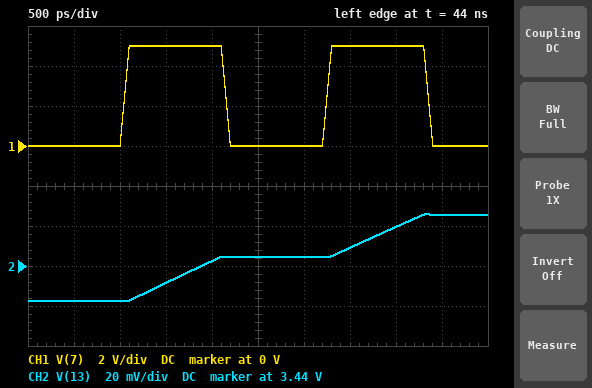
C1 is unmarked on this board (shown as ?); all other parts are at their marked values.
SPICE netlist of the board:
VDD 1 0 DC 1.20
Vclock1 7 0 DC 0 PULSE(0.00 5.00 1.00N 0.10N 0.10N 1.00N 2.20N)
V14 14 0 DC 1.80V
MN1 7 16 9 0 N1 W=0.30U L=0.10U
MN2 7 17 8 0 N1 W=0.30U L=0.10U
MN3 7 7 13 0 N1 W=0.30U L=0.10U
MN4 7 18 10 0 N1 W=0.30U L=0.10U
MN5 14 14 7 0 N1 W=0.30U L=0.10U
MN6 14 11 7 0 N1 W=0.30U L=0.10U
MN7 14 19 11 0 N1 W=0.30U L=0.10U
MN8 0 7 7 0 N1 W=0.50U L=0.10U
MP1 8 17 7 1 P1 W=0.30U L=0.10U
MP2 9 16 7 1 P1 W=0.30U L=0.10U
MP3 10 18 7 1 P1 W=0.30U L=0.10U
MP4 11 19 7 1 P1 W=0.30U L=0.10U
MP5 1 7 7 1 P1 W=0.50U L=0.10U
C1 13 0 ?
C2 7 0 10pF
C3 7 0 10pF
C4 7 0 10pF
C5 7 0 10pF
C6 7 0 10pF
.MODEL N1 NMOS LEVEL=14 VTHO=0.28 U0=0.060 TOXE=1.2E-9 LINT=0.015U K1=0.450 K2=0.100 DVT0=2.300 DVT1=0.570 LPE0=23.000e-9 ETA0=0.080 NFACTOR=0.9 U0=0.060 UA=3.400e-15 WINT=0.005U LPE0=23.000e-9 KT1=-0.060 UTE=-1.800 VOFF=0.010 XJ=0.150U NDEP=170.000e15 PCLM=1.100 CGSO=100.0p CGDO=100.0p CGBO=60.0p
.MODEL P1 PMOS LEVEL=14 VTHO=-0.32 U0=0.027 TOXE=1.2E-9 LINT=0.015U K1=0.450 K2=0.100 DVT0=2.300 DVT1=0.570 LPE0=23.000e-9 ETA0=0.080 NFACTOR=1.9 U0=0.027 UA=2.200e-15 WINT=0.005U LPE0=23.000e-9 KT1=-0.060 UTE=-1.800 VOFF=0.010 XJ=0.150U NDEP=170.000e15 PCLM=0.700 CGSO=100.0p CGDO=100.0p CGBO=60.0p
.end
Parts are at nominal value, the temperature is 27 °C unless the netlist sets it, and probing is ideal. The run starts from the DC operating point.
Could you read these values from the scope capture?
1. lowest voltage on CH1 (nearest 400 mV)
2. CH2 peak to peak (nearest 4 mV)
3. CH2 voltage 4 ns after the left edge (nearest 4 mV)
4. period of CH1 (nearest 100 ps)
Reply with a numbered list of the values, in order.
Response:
1. 0 V
2. 44 mV
3. 3.460 V
4. 2.2 ns
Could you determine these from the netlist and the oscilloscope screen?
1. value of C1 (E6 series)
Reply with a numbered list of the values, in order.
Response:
1. 15 pF
